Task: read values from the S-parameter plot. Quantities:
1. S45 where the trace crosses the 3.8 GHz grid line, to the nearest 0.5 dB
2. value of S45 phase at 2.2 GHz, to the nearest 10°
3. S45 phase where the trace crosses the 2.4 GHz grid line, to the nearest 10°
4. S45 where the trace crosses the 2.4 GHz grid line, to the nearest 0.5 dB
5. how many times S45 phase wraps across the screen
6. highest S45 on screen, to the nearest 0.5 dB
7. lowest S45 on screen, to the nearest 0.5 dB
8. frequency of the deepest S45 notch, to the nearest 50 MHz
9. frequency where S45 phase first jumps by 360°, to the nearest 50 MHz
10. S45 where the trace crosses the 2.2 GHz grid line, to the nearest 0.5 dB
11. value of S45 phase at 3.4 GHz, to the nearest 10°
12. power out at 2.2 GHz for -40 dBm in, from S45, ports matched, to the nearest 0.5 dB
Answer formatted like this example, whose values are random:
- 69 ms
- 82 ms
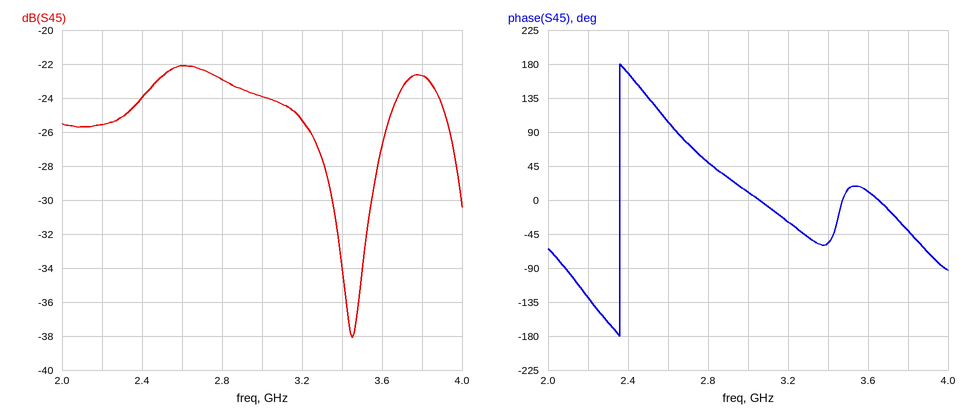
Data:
- -22.5 dB
- -130°
- 170°
- -24.0 dB
- 1
- -22.0 dB
- -38.0 dB
- 3.45 GHz
- 2.35 GHz
- -25.5 dB
- -60°
- -65.5 dBm
